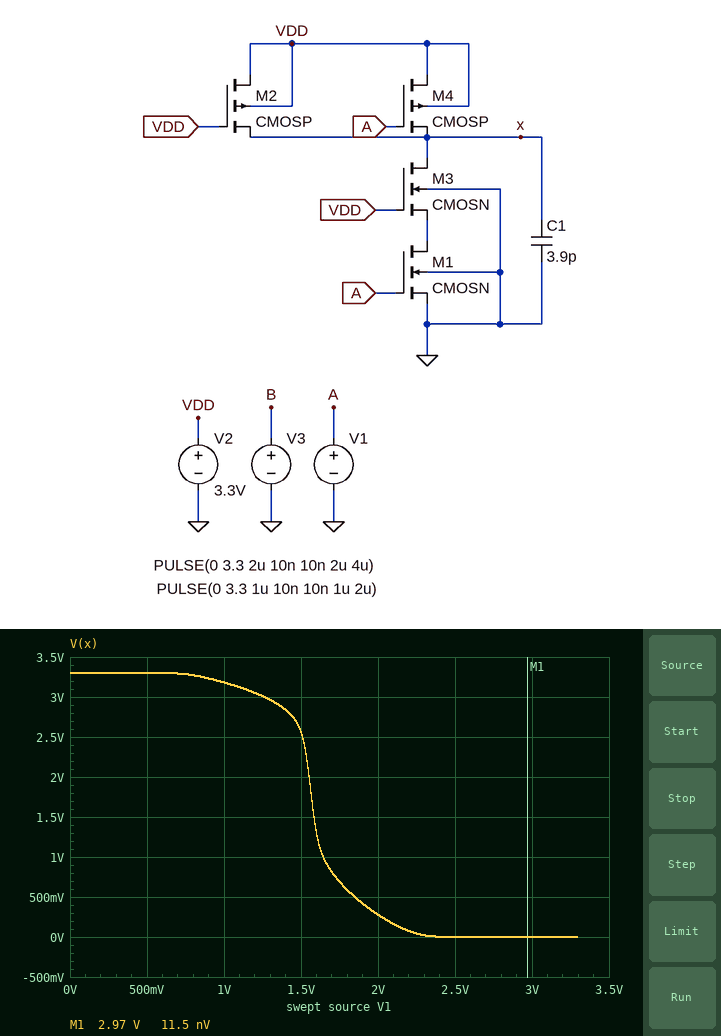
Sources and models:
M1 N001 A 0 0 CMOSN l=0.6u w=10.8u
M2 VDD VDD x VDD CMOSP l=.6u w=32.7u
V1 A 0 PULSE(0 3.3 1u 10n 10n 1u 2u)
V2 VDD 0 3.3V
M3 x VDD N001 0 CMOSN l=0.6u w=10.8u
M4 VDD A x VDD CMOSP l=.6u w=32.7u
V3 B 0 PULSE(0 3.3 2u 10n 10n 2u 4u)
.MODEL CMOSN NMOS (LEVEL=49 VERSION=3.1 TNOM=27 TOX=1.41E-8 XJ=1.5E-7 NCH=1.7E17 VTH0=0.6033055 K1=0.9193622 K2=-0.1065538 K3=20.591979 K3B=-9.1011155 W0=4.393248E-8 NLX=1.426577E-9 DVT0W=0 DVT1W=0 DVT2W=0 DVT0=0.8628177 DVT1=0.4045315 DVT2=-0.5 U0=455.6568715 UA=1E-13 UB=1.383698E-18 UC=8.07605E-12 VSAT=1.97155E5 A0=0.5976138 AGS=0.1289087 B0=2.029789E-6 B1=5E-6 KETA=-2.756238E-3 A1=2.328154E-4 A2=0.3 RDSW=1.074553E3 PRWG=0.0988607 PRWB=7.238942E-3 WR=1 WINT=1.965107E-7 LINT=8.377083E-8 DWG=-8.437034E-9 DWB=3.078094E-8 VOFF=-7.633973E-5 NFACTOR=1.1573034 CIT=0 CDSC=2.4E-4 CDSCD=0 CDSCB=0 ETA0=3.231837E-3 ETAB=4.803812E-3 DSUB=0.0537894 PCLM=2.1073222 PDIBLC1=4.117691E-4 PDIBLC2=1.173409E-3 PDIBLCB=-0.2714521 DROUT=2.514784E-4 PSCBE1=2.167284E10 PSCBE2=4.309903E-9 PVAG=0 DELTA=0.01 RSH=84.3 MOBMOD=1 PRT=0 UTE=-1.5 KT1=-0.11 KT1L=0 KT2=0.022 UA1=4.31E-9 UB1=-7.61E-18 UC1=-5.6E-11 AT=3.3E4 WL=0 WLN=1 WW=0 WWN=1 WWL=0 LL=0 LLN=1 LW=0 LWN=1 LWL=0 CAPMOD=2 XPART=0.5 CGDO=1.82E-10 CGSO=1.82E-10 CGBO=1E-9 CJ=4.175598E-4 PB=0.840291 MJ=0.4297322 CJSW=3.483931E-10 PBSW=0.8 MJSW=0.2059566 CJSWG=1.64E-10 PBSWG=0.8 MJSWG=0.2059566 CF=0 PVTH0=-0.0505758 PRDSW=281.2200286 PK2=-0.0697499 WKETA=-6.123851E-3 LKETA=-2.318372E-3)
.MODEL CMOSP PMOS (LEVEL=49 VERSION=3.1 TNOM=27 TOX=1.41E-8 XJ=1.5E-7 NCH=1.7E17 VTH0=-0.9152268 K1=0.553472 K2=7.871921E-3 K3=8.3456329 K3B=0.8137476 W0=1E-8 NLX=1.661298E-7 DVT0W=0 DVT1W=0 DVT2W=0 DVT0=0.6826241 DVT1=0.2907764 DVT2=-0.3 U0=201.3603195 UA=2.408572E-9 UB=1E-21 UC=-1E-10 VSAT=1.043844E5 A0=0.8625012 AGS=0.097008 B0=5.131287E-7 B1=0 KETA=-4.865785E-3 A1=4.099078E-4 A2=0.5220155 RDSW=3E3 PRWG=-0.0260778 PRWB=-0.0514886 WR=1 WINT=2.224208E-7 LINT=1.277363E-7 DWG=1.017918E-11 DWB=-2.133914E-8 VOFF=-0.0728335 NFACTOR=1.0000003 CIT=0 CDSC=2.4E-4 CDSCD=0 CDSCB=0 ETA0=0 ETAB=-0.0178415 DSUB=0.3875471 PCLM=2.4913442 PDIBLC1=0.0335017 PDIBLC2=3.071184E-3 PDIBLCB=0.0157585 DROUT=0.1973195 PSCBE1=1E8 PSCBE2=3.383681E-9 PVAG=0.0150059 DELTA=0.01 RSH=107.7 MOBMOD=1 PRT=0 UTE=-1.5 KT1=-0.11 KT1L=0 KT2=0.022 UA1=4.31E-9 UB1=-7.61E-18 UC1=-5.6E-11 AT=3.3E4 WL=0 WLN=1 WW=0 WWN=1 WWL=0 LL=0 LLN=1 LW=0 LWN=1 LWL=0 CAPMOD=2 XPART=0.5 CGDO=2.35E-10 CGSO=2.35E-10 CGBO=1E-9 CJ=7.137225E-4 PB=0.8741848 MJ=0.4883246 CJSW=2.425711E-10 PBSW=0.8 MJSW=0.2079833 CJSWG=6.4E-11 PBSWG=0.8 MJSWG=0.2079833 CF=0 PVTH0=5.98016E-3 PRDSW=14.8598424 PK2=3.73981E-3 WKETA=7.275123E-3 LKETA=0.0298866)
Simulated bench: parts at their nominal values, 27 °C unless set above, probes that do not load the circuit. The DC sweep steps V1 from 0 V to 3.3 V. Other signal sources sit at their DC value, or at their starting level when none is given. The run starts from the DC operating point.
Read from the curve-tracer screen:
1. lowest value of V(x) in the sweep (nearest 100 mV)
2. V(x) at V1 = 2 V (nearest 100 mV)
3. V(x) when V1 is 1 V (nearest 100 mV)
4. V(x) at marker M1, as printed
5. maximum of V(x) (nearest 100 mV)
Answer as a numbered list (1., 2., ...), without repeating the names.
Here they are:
1. 0 V
2. 300 mV
3. 3.2 V
4. 11.5 nV
5. 3.3 V
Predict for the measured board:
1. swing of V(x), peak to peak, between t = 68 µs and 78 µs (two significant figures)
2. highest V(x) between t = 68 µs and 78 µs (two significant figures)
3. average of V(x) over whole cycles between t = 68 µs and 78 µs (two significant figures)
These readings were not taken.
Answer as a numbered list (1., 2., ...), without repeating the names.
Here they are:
1. 3.3 V
2. 3.3 V
3. 1.6 V
